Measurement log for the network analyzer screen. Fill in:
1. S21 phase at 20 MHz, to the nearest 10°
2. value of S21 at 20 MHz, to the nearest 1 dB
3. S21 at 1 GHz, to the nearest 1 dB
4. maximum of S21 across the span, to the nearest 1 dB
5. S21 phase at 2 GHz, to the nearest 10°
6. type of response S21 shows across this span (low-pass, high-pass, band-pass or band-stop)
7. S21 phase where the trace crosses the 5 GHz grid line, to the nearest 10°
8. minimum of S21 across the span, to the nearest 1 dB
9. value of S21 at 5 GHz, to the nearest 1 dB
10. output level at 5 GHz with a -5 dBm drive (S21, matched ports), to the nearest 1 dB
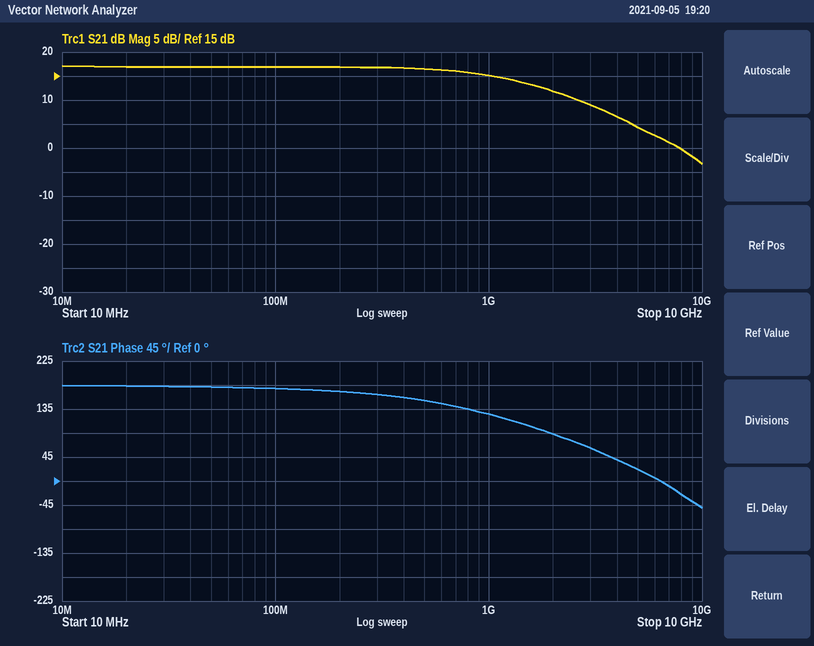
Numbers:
180°
17 dB
15 dB
17 dB
90°
low-pass
20°
-3 dB
4 dB
-1 dBm
